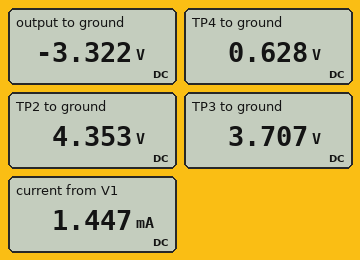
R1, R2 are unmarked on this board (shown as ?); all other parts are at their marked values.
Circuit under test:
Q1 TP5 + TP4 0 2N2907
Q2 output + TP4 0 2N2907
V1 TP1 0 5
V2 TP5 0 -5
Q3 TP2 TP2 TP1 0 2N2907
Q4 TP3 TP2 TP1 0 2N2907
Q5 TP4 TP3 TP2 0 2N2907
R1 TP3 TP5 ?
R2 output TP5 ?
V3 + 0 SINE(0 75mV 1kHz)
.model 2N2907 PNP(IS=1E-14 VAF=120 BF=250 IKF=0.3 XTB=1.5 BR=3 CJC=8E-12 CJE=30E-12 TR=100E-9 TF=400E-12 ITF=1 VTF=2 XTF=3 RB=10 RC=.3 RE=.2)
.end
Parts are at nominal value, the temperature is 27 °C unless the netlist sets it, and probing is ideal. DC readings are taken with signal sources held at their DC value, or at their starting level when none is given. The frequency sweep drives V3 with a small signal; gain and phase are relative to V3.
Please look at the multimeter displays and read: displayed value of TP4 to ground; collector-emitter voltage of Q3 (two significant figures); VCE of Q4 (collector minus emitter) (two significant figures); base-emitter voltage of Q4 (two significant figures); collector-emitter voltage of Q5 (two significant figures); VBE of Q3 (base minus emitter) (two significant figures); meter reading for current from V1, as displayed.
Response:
0.628 V
-650 mV
-1.3 V
-650 mV
-3.7 V
-650 mV
1.447 mA
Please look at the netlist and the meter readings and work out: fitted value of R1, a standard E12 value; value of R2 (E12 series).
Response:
12 kΩ
4.7 kΩ
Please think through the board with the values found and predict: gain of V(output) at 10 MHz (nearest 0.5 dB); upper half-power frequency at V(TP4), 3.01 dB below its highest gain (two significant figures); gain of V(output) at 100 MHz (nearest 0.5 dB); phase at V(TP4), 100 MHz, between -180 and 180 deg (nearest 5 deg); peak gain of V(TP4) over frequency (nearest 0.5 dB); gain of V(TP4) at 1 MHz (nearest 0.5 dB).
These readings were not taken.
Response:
-13.0 dB
3.5 GHz
0 dB
0 deg
0 dB
0 dB
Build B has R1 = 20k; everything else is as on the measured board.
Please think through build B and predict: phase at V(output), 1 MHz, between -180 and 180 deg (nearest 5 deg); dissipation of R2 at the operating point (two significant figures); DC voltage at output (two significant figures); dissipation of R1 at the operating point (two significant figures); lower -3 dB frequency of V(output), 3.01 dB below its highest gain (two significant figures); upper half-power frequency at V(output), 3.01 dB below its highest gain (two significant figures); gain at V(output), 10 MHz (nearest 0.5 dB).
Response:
-140 deg
220 µW
-4.0 V
3.8 mW
20 MHz
4.1 GHz
-9.0 dB
